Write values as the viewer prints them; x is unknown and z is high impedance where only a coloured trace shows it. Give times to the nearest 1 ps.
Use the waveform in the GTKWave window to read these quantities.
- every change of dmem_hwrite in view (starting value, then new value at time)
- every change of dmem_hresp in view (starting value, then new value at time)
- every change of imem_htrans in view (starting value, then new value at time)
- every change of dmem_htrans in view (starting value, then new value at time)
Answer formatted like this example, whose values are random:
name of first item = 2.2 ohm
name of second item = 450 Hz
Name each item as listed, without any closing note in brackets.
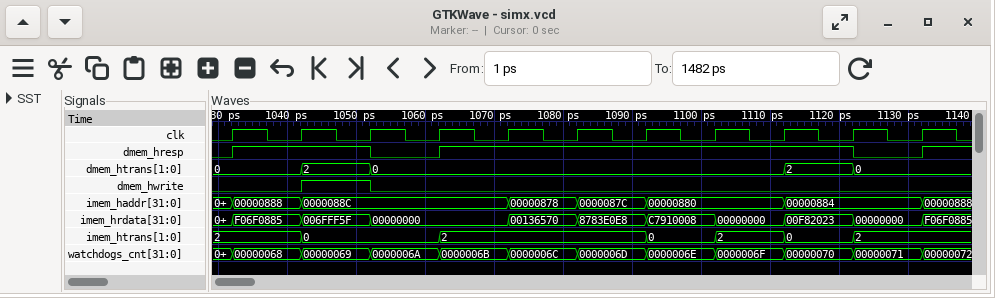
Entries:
every change of dmem_hwrite in view = 0, 1 at 1042 ps, 0 at 1052 ps
every change of dmem_hresp in view = 0, 1 at 1032 ps, 0 at 1052 ps, 1 at 1062 ps, 0 at 1122 ps, 1 at 1132 ps
every change of imem_htrans in view = 2, 0 at 1042 ps, 2 at 1062 ps, 0 at 1092 ps, 2 at 1102 ps, 0 at 1112 ps, 2 at 1122 ps
every change of dmem_htrans in view = 0, 2 at 1042 ps, 0 at 1052 ps, 2 at 1112 ps, 0 at 1122 ps
